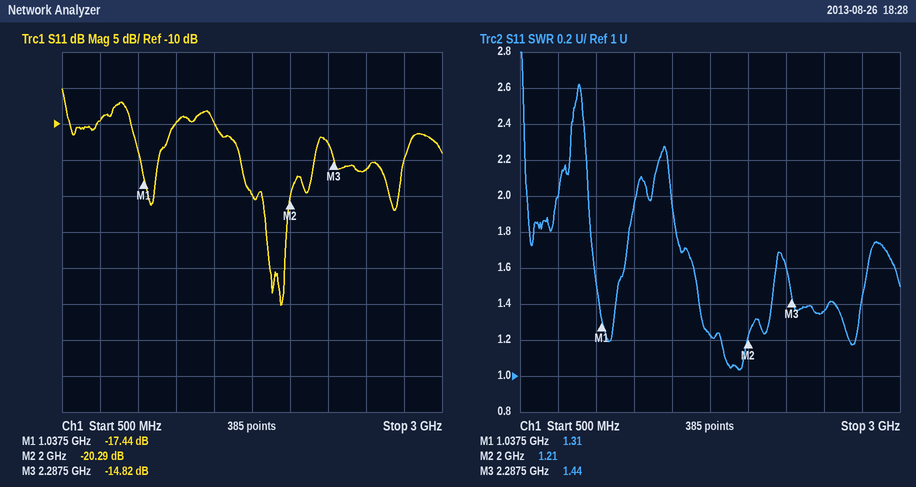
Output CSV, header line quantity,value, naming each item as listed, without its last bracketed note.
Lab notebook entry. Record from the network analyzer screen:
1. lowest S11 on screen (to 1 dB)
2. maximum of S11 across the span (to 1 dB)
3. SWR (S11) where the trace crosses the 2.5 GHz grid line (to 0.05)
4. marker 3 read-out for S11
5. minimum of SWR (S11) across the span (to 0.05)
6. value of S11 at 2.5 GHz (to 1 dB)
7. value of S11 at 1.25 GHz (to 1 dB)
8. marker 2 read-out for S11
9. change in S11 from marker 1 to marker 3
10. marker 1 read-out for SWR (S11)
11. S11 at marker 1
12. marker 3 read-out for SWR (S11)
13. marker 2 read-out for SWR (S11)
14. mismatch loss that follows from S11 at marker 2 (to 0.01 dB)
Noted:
quantity,value
lowest S11 on screen,-35 dB
maximum of S11 across the span,-5 dB
SWR (S11) where the trace crosses the 2.5 GHz grid line,1.35
marker 3 read-out for S11,-14.82 dB
minimum of SWR (S11) across the span,1.05
value of S11 at 2.5 GHz,-16 dB
value of S11 at 1.25 GHz,-10 dB
marker 2 read-out for S11,-20.29 dB
change in S11 from marker 1 to marker 3,2.62 dB
marker 1 read-out for SWR,1.31
S11 at marker 1,-17.44 dB
marker 3 read-out for SWR,1.44
marker 2 read-out for SWR,1.21
mismatch loss that follows from S11 at marker 2,0.04 dB
